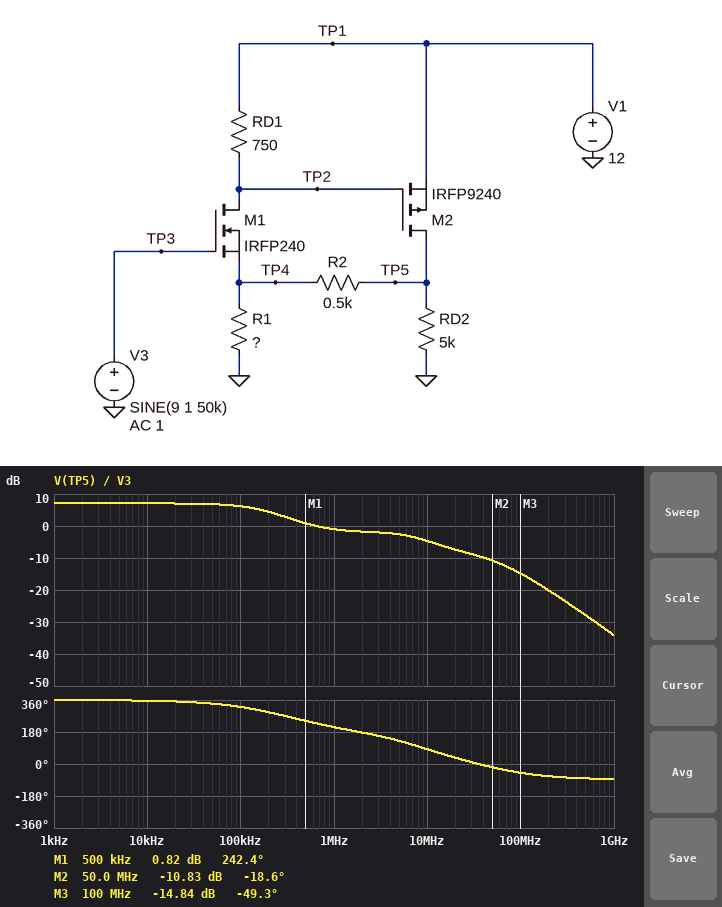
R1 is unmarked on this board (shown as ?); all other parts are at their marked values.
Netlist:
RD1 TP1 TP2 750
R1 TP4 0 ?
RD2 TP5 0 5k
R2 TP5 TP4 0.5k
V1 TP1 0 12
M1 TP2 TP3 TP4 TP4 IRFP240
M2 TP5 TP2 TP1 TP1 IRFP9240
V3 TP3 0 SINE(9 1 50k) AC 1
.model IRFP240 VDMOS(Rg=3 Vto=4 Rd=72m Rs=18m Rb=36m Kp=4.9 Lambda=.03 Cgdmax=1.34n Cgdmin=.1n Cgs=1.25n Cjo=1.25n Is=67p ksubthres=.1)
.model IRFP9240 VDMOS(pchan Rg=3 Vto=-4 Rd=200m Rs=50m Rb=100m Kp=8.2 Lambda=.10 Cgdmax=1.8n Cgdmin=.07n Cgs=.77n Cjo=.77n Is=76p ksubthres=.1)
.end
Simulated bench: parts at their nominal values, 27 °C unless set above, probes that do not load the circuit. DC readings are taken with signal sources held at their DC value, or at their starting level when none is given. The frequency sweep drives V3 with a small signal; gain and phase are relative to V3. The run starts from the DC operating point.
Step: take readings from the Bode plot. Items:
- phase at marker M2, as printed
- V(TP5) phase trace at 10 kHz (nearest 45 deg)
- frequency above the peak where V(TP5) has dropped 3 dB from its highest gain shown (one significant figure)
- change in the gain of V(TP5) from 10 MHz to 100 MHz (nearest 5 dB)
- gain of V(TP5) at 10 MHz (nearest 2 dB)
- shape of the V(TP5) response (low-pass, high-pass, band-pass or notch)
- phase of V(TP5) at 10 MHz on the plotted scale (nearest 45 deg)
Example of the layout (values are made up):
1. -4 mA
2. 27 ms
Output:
1. -18.6 deg
2. 360 deg
3. 200 kHz
4. -10 dB
5. -4 dB
6. low-pass
7. 90 deg
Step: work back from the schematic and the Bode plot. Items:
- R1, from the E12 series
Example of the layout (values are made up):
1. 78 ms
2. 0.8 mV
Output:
1. 390 Ω
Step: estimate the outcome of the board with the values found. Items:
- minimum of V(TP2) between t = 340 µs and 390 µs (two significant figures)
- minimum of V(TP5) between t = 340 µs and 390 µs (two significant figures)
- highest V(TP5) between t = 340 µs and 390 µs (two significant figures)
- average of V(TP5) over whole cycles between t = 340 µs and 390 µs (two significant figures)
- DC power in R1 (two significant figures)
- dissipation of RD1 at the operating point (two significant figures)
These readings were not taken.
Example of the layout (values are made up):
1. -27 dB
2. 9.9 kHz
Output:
1. 8.0 V
2. 6.7 V
3. 11 V
4. 8.9 V
5. 66 mW
6. 21 mW
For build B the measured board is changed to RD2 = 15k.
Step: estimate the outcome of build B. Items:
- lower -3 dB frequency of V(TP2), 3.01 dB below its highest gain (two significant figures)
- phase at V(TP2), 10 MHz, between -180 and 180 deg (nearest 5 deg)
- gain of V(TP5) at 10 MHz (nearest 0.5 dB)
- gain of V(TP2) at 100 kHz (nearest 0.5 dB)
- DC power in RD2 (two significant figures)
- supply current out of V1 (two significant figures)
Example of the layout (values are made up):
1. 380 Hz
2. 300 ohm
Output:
1. 5.1 MHz
2. 30 deg
3. -5.0 dB
4. -29.5 dB
5. 5.3 mW
6. 14 mA
